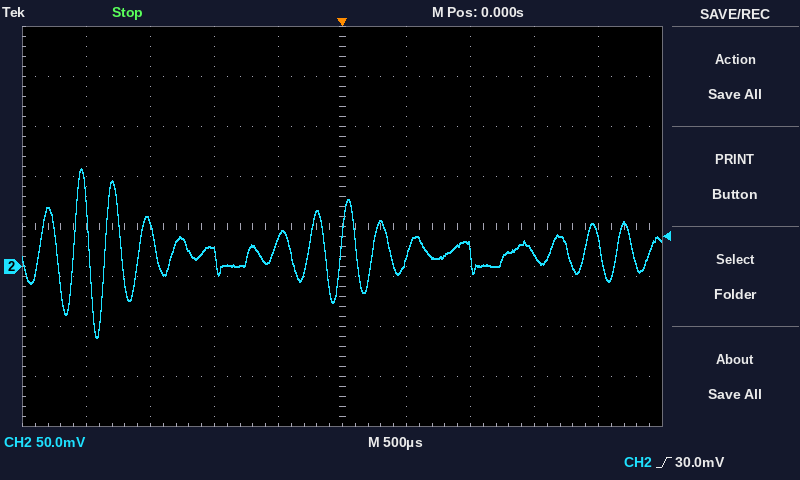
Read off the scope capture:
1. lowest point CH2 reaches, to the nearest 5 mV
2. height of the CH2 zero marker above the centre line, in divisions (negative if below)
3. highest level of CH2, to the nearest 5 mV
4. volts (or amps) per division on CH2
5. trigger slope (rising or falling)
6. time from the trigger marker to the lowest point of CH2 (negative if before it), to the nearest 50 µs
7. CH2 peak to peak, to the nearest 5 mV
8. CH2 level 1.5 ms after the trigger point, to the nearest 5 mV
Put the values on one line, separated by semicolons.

-70 mV; -0.8 div; 100 mV; 50 mV; rising; -1.90 ms; 170 mV; 10 mV
